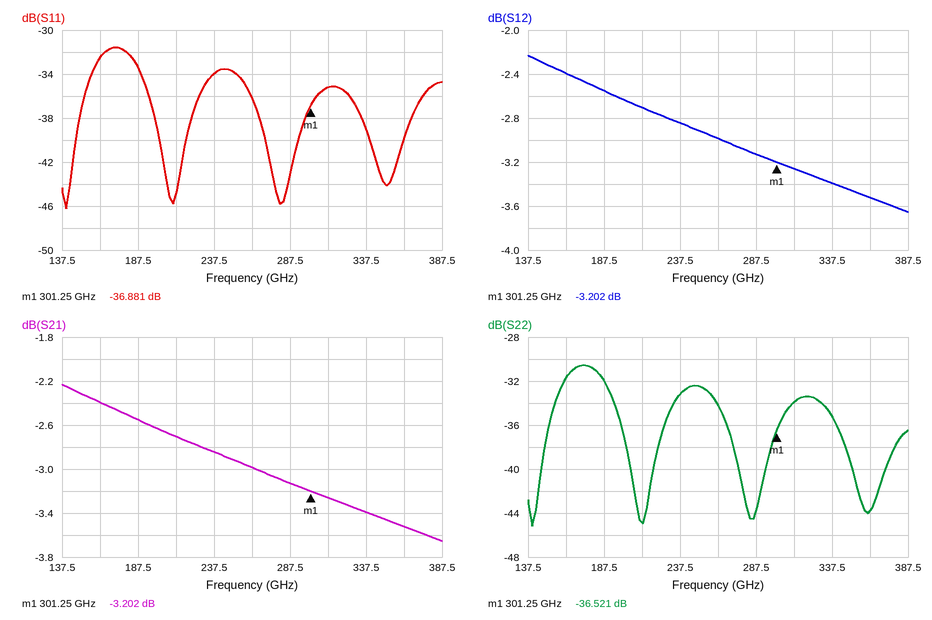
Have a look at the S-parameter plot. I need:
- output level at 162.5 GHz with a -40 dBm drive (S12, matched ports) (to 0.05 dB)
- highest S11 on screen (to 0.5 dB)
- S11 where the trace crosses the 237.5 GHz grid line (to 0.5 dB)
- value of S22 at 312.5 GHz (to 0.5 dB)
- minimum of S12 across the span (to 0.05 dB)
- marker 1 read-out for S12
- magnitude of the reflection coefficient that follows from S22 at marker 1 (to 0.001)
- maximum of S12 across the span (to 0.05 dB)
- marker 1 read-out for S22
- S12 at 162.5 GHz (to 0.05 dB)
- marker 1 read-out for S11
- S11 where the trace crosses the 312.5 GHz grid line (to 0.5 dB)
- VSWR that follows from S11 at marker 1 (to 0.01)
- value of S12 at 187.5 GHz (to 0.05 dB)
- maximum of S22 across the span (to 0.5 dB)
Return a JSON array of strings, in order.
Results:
["-42.40 dBm", "-31.5 dB", "-34.0 dB", "-34.0 dB", "-3.65 dB", "-3.202 dB", "0.015", "-2.25 dB", "-36.521 dB", "-2.40 dB", "-36.881 dB", "-35.0 dB", "1.03", "-2.55 dB", "-30.5 dB"]
